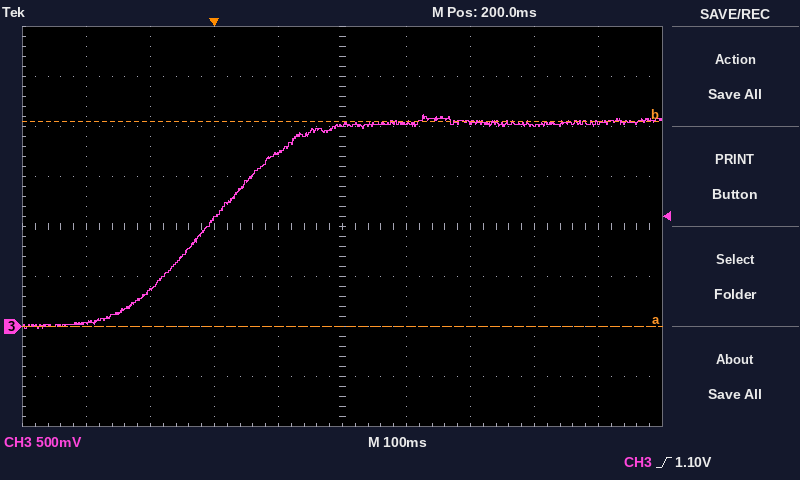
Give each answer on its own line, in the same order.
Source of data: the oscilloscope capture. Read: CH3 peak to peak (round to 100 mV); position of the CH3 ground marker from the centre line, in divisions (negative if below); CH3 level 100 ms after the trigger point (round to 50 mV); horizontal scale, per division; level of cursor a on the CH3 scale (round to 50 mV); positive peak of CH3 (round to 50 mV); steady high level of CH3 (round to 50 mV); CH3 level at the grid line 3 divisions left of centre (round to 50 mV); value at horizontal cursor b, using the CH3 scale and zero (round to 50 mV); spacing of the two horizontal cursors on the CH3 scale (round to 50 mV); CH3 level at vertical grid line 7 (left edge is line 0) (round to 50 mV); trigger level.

2.10 V
-2.0 div
1.75 V
100 ms
0 mV
2.10 V
2.05 V
350 mV
2.05 V
2.05 V
2.05 V
1.10 V
